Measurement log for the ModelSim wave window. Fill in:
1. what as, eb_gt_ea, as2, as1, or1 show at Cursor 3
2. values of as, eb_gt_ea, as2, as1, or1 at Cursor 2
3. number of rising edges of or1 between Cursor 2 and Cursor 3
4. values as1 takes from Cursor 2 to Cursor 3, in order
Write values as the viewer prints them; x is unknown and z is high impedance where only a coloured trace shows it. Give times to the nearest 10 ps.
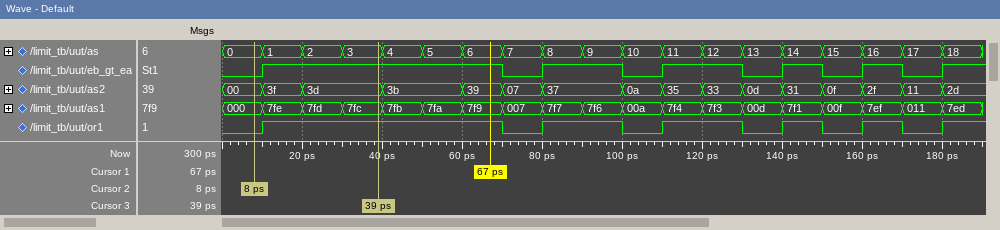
as=3, eb_gt_ea=1, as2=3d, as1=7fc, or1=1
as=0, eb_gt_ea=0, as2=00, as1=000, or1=0
1
000, 7fe, 7fd, 7fc
